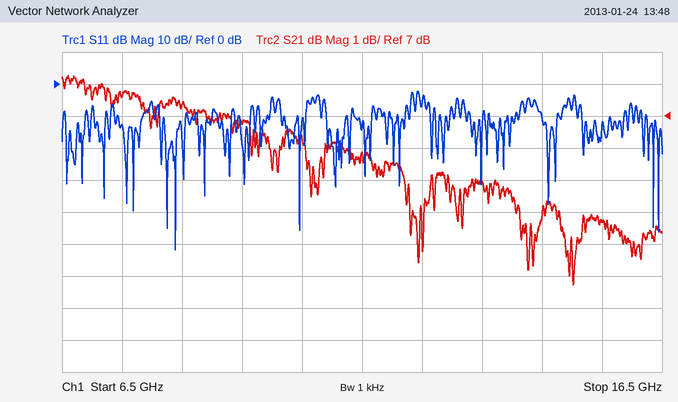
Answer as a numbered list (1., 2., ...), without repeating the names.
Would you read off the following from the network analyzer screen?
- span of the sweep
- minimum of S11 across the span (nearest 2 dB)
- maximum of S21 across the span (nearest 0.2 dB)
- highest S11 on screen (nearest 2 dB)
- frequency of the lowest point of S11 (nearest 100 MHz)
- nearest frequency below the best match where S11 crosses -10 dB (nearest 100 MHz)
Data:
1. 10 GHz
2. -52 dB
3. 8.2 dB
4. -2 dB
5. 8.4 GHz
6. 8.1 GHz
